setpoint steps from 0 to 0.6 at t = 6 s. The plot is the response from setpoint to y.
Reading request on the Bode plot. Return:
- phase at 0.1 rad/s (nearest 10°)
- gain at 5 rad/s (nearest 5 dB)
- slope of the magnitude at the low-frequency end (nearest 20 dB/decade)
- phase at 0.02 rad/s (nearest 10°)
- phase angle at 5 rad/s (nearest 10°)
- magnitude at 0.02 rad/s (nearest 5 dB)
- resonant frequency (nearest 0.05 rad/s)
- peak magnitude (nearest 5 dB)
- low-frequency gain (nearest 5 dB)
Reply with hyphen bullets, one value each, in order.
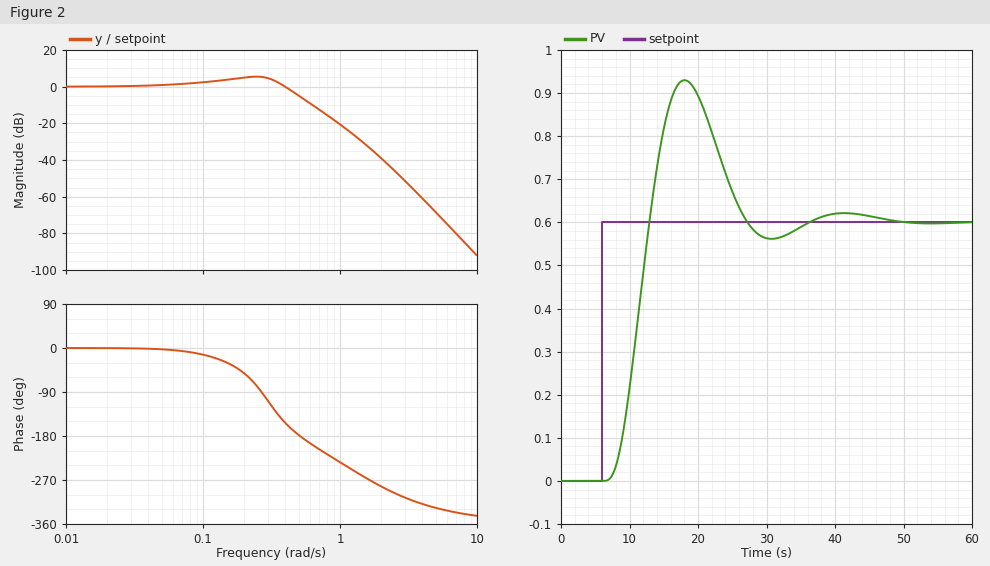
- -10°
- -70 dB
- 0 dB/decade
- 0°
- -330°
- 0 dB
- 0.25 rad/s
- 5 dB
- 0 dB
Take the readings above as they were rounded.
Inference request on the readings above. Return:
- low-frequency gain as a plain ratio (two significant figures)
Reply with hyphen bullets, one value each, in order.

- 1.0
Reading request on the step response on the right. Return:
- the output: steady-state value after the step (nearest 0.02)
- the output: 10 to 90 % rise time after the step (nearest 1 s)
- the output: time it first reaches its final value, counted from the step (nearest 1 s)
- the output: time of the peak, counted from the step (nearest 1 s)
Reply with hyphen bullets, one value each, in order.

- 0.60
- 4 s
- 7 s
- 12 s
